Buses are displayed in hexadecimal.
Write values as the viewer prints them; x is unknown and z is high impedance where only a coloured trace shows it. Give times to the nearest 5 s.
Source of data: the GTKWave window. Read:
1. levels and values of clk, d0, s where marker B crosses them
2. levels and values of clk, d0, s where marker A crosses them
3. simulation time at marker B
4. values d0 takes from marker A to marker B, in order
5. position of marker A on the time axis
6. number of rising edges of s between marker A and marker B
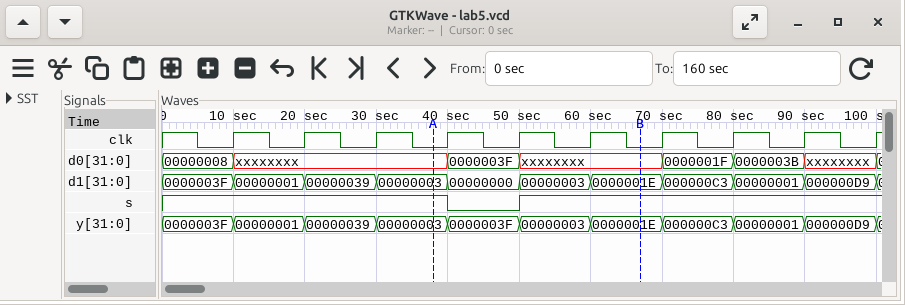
clk=0, d0=xxxxxxxx, s=1
clk=0, d0=xxxxxxxx, s=1
65 s
xxxxxxxx, 0000003F, xxxxxxxx
40 s
1
